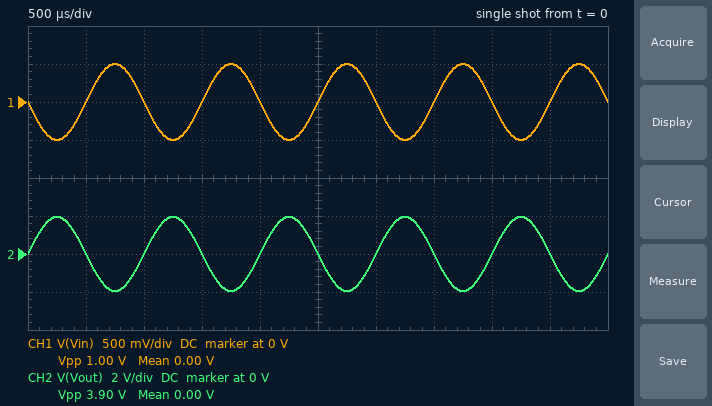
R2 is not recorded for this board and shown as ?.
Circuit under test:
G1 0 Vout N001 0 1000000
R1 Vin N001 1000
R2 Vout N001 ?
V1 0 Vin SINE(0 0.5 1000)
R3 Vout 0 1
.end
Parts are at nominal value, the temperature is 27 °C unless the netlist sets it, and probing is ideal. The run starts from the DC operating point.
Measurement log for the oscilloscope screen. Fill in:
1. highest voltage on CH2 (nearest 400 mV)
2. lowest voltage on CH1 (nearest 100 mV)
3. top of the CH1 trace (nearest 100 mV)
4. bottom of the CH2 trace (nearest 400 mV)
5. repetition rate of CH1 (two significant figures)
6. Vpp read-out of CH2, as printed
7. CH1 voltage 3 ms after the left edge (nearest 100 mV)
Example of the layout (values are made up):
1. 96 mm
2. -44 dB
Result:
1. 2.0 V
2. -500 mV
3. 500 mV
4. -2.0 V
5. 1.0 kHz
6. 3.90 V
7. 0 V
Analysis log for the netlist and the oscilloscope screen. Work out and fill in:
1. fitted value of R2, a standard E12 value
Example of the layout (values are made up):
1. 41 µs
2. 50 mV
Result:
1. 3.9 kΩ
